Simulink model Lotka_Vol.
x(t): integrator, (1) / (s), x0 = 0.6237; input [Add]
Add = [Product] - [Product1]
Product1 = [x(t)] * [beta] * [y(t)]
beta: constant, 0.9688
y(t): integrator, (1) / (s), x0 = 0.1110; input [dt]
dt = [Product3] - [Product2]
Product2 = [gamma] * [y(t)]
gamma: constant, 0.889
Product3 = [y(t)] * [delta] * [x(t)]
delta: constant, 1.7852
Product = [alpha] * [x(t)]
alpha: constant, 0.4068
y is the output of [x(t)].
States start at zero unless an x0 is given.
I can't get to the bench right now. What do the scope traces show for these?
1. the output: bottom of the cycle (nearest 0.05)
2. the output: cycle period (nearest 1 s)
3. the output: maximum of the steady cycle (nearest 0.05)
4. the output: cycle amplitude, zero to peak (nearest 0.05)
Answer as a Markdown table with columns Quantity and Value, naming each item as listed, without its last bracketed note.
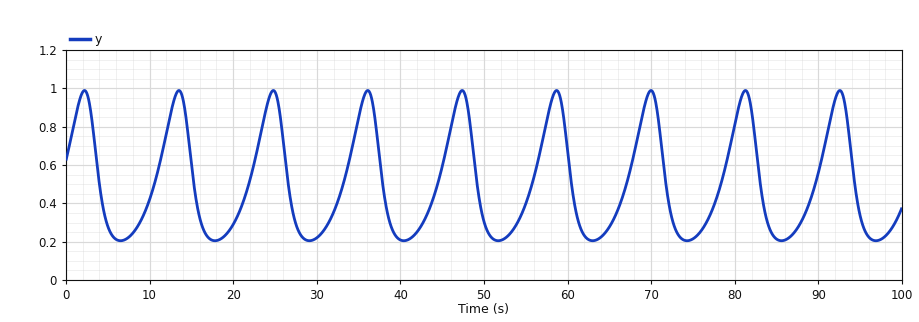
| Quantity | Value |
|---|---|
| the output: bottom of the cycle | 0.20 |
| the output: cycle period | 11 s |
| the output: maximum of the steady cycle | 1.00 |
| the output: cycle amplitude, zero to peak | 0.40 |
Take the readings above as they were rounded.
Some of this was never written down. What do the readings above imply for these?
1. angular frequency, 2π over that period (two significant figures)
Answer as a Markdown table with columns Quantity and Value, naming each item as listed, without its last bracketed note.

| Quantity | Value |
|---|---|
| angular frequency, 2π over that period | 0.57 rad/s |
